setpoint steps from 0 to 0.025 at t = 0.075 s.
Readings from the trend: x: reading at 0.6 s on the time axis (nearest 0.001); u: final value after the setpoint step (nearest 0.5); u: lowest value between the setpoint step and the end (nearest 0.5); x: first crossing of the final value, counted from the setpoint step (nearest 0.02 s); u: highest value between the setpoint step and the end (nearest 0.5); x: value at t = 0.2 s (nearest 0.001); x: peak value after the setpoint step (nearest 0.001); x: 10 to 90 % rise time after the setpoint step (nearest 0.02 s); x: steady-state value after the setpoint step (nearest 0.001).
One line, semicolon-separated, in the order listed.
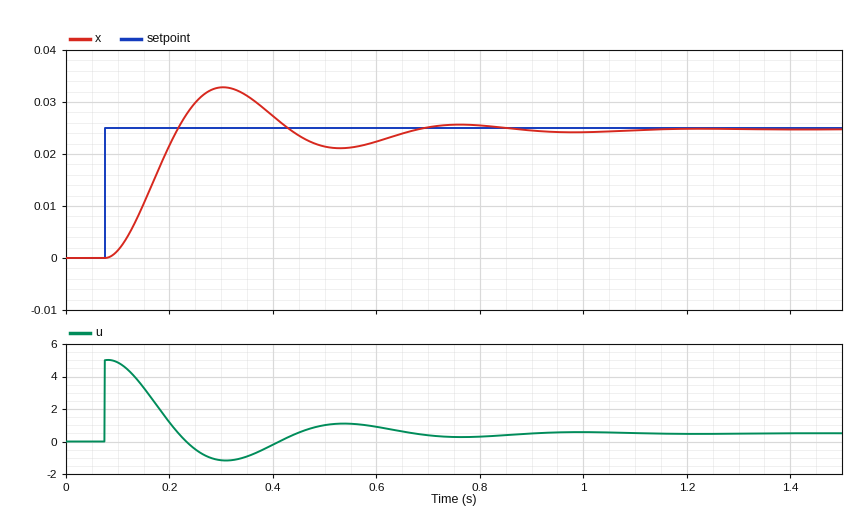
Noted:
0.022; 0.5; -1.0; 0.14 s; 5.0; 0.022; 0.033; 0.10 s; 0.025
